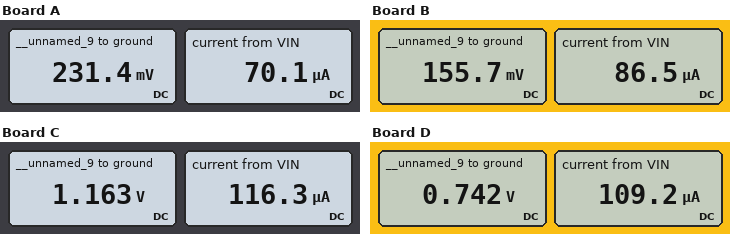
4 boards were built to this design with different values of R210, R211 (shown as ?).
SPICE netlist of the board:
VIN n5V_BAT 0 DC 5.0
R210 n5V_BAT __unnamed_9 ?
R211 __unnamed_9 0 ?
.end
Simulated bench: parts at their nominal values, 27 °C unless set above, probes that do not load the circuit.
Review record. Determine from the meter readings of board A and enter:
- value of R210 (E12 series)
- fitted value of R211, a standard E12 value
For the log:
68 kΩ
3.3 kΩ
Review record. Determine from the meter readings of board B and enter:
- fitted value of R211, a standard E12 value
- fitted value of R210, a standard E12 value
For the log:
1.8 kΩ
56 kΩ
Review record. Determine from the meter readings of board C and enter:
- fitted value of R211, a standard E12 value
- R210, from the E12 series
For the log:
10 kΩ
33 kΩ
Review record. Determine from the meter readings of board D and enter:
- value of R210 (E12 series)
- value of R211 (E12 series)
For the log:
39 kΩ
6.8 kΩ
